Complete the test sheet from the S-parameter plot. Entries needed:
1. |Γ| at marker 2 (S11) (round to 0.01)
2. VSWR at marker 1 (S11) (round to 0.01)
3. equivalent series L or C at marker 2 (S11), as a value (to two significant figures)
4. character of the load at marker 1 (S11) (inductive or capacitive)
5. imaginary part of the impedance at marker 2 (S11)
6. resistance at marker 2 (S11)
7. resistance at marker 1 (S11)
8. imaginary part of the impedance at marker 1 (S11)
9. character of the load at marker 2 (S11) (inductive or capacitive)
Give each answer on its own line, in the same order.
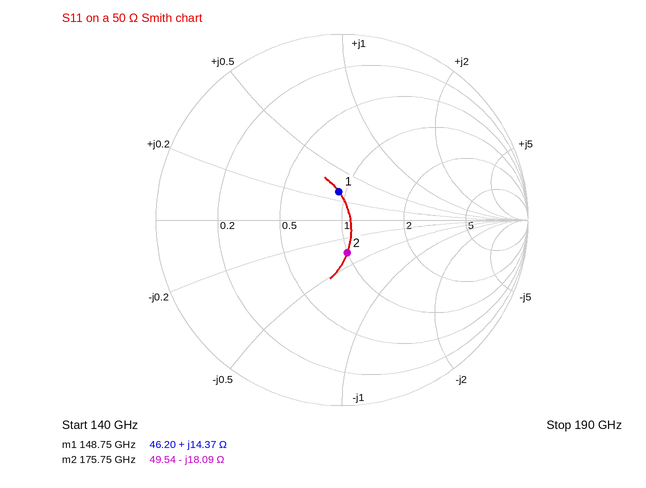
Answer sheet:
0.18
1.36
50 fF
inductive
-18.09 Ω
49.54 Ω
46.20 Ω
+14.37 Ω
capacitive
